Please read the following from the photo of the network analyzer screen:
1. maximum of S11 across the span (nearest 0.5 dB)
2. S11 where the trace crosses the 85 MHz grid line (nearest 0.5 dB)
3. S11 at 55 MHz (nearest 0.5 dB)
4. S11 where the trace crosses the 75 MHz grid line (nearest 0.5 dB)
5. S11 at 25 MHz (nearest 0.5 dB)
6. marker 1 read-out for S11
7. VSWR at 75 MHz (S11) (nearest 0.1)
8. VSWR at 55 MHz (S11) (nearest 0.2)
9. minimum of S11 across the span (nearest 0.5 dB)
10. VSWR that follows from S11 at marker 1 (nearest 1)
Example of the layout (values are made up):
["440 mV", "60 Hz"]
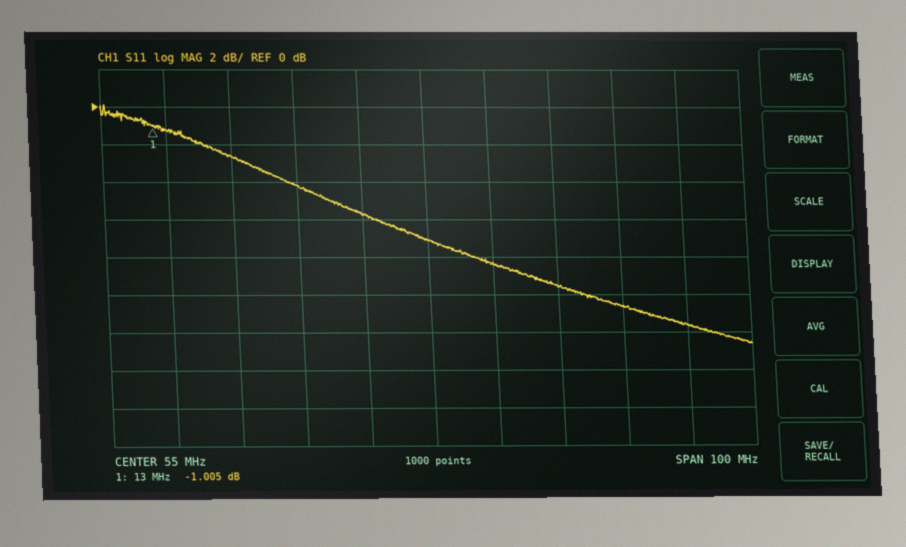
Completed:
["0.0 dB", "-10.5 dB", "-7.0 dB", "-9.5 dB", "-2.5 dB", "-1.005 dB", "2.0", "2.6", "-12.5 dB", "17"]
